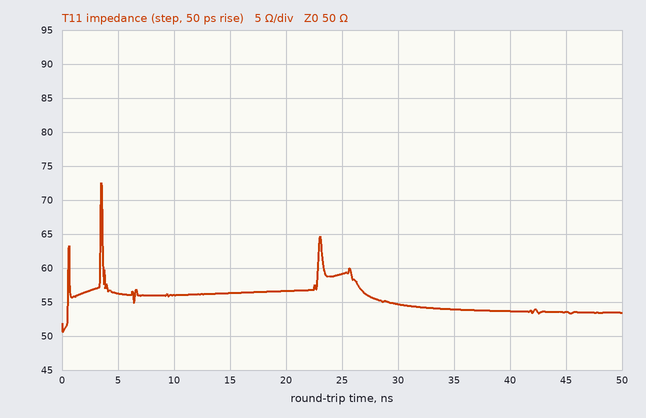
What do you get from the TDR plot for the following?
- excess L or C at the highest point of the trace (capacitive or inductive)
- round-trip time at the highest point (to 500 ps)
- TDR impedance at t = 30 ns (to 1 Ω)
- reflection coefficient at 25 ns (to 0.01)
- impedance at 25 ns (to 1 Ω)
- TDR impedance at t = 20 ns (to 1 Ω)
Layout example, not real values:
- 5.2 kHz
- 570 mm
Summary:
- inductive
- 3.5 ns
- 55 Ω
- +0.08
- 59 Ω
- 57 Ω
